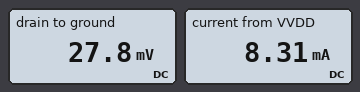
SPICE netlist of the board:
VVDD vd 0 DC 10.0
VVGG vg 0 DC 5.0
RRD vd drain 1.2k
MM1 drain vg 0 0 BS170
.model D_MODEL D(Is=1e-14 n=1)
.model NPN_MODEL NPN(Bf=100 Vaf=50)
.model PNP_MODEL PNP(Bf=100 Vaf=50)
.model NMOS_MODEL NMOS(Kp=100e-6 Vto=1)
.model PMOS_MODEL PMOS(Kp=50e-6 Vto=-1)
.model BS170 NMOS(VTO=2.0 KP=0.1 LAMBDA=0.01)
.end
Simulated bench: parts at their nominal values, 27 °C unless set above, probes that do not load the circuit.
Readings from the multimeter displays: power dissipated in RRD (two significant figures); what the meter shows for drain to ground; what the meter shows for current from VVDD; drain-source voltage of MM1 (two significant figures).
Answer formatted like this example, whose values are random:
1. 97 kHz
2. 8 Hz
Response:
1. 83 mW
2. 27.8 mV
3. 8.31 mA
4. 28 mV
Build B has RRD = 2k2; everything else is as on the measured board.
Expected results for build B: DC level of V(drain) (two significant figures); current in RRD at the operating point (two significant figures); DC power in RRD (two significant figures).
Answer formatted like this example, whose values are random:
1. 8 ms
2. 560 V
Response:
1. 15 mV
2. 4.5 mA
3. 45 mW
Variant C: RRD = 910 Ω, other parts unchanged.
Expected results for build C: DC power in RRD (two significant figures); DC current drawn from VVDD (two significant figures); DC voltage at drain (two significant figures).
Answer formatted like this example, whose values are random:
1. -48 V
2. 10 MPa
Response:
1. 110 mW
2. 11 mA
3. 37 mV
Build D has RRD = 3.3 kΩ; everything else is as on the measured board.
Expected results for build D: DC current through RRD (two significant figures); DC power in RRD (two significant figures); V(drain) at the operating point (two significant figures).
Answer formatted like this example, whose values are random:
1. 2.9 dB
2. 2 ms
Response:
1. 3.0 mA
2. 30 mW
3. 10 mV
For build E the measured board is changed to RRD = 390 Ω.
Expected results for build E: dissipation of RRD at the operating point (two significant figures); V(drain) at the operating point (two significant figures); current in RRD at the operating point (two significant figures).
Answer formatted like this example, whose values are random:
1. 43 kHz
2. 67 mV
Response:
1. 250 mW
2. 86 mV
3. 25 mA
